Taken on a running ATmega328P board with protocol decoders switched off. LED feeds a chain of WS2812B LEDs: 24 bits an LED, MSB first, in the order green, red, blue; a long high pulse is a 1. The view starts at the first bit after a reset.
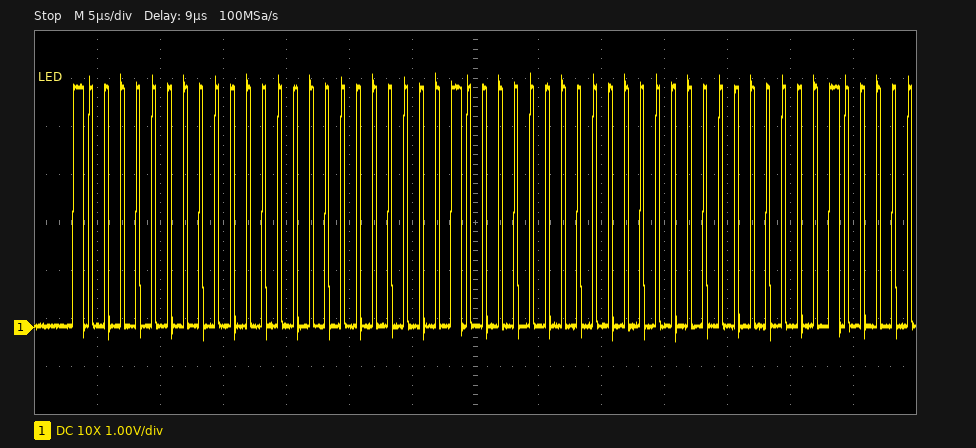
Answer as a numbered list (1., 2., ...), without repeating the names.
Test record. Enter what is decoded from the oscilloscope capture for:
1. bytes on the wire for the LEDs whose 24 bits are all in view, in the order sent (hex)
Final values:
1. 80 00 00 80 00 00
